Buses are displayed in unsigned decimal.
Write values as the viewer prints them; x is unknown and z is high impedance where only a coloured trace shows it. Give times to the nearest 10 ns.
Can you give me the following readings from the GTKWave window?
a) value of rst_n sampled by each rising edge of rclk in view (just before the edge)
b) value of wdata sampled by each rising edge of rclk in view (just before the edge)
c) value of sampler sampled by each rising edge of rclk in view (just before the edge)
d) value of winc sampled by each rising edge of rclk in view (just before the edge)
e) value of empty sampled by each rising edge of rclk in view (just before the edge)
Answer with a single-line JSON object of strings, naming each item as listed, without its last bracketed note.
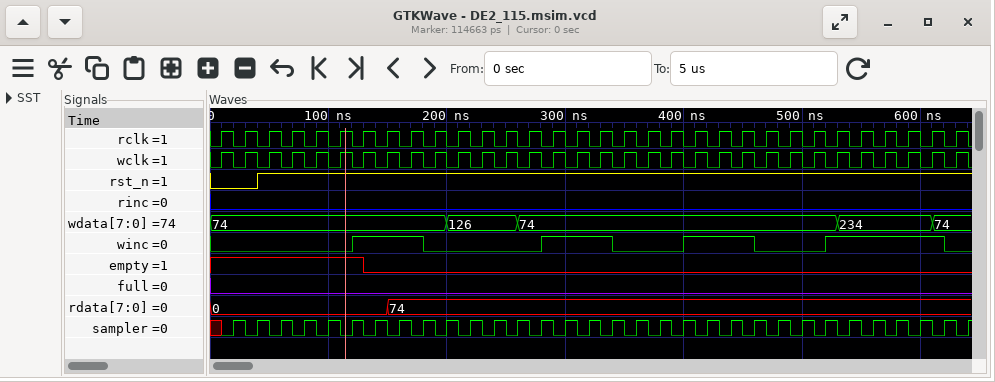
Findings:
{"value of rst_n sampled by each rising edge of rclk in view": "0 0 1 1 1 1 1 1 1 1 1 1 1 1 1 1 1 1 1 1 1 1 1 1 1 1 1 1 1 1 1 1", "value of wdata sampled by each rising edge of rclk in view": "74, 74, 74, 74, 74, 74, 74, 74, 74, 74, 126, 126, 126, 74, 74, 74, 74, 74, 74, 74, 74, 74, 74, 74, 74, 74, 74, 234, 234, 234, 234, 74", "value of sampler sampled by each rising edge of rclk in view": "x 1 1 1 1 1 1 1 1 1 1 1 1 1 1 1 1 1 1 1 1 1 1 1 1 1 1 1 1 1 1 1", "value of winc sampled by each rising edge of rclk in view": "0 0 0 0 0 0 1 1 1 0 0 0 0 0 1 1 1 0 0 0 1 1 1 0 0 0 1 1 1 1 1 0", "value of empty sampled by each rising edge of rclk in view": "1 1 1 1 1 1 1 0 0 0 0 0 0 0 0 0 0 0 0 0 0 0 0 0 0 0 0 0 0 0 0 0"}
